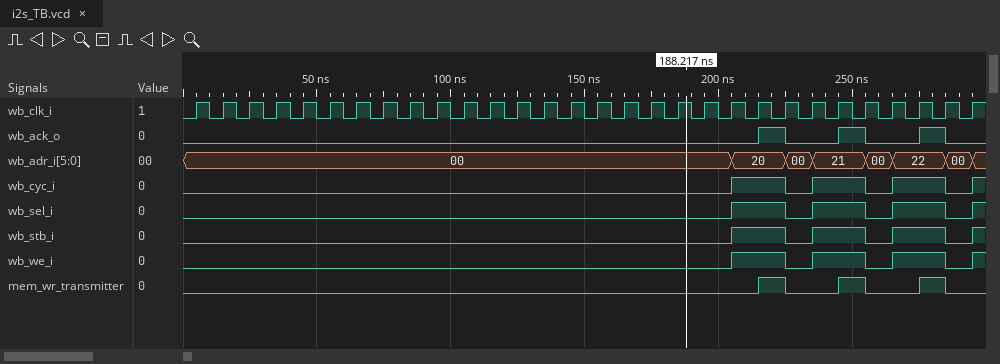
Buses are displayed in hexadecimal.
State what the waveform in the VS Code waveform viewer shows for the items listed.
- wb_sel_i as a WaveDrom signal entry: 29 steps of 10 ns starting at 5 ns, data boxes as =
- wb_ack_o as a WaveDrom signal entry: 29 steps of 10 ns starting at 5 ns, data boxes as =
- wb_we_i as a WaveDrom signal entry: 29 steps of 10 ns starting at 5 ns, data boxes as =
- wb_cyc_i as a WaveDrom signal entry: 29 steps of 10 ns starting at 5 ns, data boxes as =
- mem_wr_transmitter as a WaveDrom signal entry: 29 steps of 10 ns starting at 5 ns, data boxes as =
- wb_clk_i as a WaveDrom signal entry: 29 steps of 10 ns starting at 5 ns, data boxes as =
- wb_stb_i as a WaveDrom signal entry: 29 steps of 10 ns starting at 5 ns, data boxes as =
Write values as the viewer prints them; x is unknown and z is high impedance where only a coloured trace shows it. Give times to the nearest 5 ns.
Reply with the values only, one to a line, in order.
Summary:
{name: 'wb_sel_i', wave: '0...................1.01.01.0'}
{name: 'wb_ack_o', wave: '0....................10.10.10'}
{name: 'wb_we_i', wave: '0...................1.01.01.0'}
{name: 'wb_cyc_i', wave: '0...................1.01.01.0'}
{name: 'mem_wr_transmitter', wave: '0....................10.10.10'}
{name: 'wb_clk_i', wave: 'p............................'}
{name: 'wb_stb_i', wave: '0...................1.01.01.0'}
